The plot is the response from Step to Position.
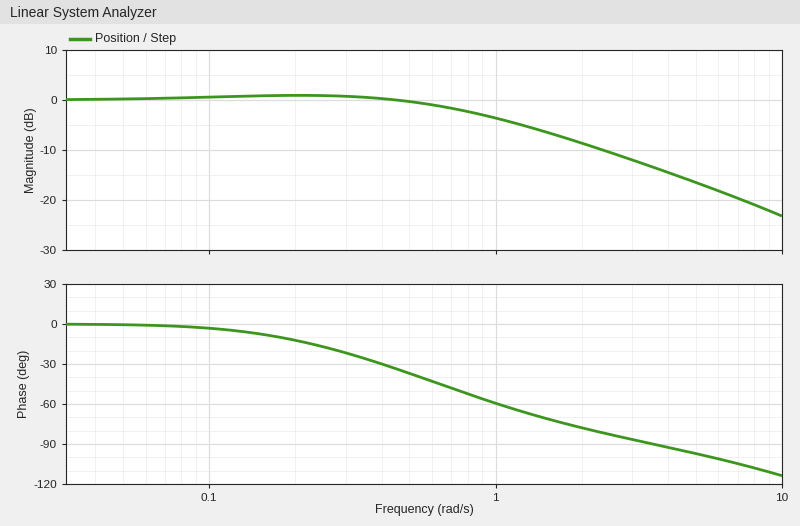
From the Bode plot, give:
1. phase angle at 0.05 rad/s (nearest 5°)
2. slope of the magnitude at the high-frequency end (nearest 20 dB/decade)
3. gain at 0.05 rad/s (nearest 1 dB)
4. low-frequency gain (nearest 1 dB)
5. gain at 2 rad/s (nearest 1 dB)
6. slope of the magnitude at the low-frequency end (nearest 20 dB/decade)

0°
-20 dB/decade
0 dB
0 dB
-9 dB
0 dB/decade
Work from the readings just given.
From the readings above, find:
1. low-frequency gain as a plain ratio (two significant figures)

1.0
